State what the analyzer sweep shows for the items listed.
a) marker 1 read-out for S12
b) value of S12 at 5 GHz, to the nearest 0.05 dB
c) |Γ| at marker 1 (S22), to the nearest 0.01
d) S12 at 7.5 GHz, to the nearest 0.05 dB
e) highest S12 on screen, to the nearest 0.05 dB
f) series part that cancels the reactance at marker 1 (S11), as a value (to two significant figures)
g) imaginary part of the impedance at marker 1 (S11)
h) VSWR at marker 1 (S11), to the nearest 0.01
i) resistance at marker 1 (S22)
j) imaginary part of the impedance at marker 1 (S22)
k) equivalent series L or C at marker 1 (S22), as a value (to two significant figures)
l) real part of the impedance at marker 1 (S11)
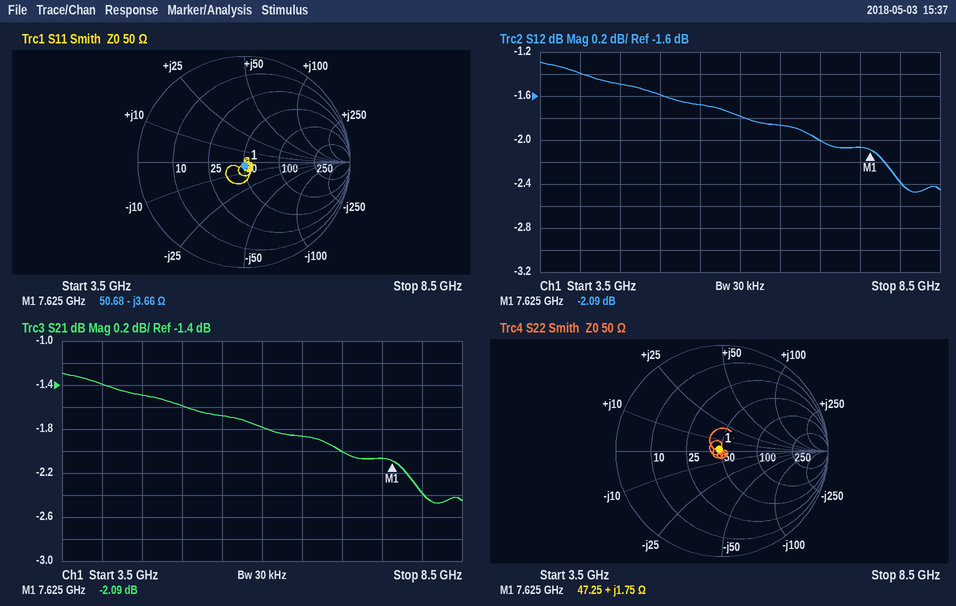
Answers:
-2.09 dB
-1.60 dB
0.03
-2.05 dB
-1.30 dB
76 pH
-3.66 Ω
1.08
47.25 Ω
+1.75 Ω
37 pH
50.68 Ω
